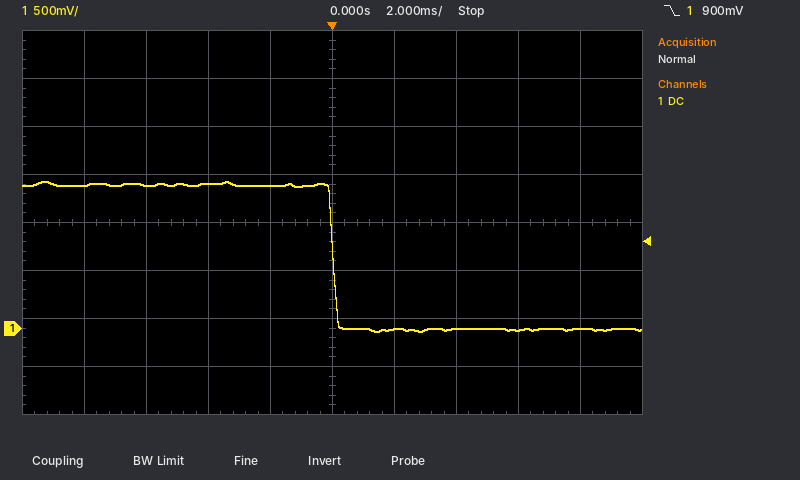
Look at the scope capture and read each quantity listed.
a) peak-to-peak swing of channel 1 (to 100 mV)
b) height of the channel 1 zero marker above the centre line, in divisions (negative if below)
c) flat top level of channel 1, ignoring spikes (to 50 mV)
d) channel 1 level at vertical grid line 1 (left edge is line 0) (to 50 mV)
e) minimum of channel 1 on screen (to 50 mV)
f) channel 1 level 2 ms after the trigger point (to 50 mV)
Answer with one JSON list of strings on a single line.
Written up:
["1.60 V", "-2.2 div", "1.50 V", "1.50 V", "-50 mV", "0 mV"]
